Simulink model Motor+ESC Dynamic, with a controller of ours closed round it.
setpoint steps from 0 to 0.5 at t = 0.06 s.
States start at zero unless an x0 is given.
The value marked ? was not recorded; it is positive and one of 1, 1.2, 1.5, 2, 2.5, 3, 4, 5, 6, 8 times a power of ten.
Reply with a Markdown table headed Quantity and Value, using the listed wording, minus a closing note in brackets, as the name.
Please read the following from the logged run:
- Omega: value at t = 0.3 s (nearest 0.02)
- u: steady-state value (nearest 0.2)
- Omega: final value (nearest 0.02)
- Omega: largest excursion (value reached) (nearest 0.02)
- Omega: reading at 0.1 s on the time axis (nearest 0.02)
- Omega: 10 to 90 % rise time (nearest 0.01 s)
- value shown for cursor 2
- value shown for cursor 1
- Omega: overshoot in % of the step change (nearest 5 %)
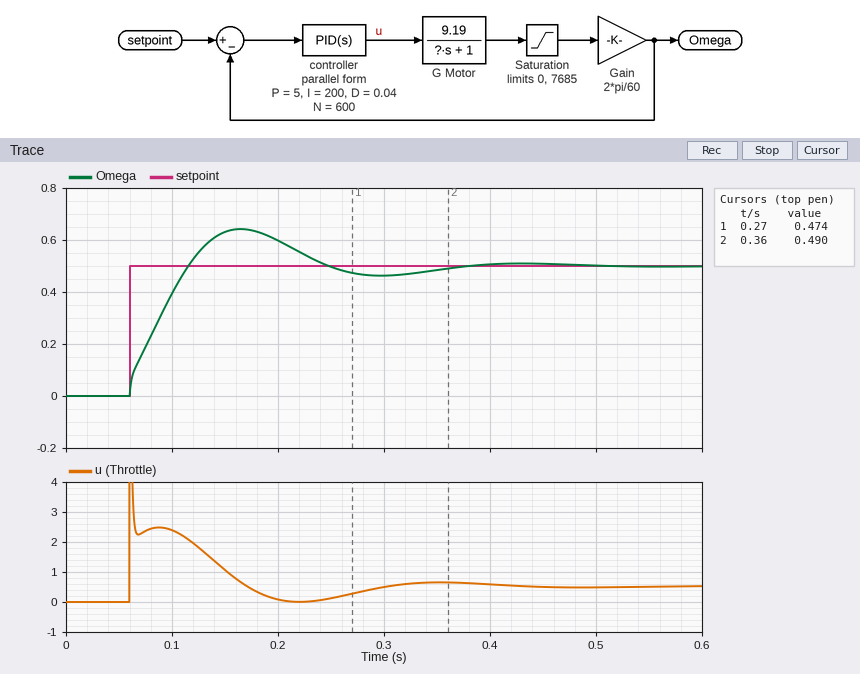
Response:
| Quantity | Value |
|---|---|
| Omega: value at t = 0.3 s | 0.46 |
| u: steady-state value | 0.6 |
| Omega: final value | 0.50 |
| Omega: largest excursion (value reached) | 0.64 |
| Omega: reading at 0.1 s on the time axis | 0.40 |
| Omega: 10 to 90 % rise time | 0.05 s |
| value shown for cursor 2 | 0.490 |
| value shown for cursor 1 | 0.474 |
| Omega: overshoot in % of the step change | 30 % |
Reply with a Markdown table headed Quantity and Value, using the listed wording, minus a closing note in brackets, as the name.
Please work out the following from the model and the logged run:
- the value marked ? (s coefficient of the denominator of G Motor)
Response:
| Quantity | Value |
|---|---|
| the value marked ? | 0.25 |
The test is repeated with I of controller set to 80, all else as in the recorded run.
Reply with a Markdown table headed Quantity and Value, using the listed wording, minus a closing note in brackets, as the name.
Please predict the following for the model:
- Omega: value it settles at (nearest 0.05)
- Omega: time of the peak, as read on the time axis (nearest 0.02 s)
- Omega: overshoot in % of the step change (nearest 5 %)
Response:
| Quantity | Value |
|---|---|
| Omega: value it settles at | 0.50 |
| Omega: time of the peak, as read on the time axis | 0.22 s |
| Omega: overshoot in % of the step change | 15 % |
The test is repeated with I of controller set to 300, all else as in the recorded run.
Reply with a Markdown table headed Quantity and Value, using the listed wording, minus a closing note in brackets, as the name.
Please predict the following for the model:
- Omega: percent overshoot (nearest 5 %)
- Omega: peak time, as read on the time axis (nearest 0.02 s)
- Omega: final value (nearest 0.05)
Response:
| Quantity | Value |
|---|---|
| Omega: percent overshoot | 35 % |
| Omega: peak time, as read on the time axis | 0.14 s |
| Omega: final value | 0.50 |
